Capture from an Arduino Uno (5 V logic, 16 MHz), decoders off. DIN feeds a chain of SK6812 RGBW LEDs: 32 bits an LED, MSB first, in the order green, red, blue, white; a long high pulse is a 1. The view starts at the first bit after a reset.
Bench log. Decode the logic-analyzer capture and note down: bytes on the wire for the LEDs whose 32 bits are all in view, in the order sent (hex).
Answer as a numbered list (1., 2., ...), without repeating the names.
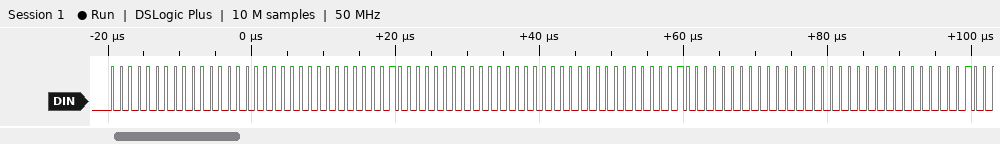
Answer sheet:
1. 00 00 00 01 00 00 00 01 00 00 00 01
